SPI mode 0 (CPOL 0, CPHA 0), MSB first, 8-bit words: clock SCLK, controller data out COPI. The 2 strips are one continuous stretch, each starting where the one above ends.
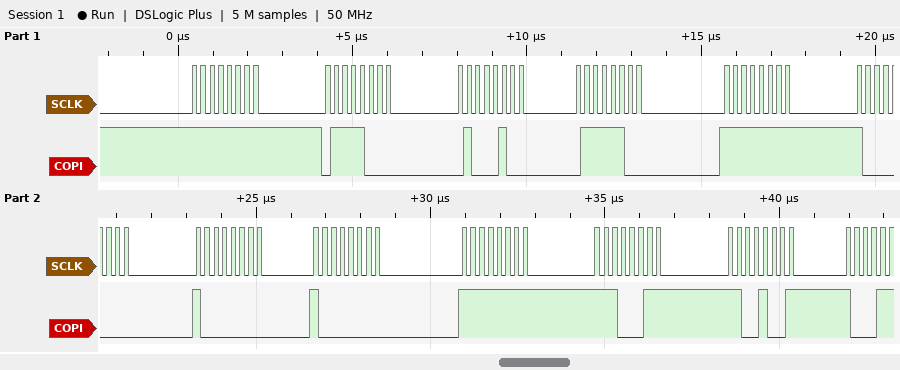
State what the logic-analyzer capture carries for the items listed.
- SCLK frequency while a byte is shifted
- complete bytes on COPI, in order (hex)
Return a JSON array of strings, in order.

["4 MHz", "FF 78 44 7C FF 80 80 80 FF E3 C9"]
